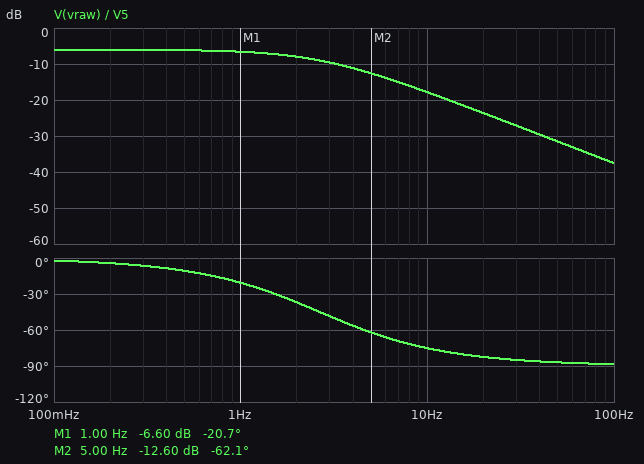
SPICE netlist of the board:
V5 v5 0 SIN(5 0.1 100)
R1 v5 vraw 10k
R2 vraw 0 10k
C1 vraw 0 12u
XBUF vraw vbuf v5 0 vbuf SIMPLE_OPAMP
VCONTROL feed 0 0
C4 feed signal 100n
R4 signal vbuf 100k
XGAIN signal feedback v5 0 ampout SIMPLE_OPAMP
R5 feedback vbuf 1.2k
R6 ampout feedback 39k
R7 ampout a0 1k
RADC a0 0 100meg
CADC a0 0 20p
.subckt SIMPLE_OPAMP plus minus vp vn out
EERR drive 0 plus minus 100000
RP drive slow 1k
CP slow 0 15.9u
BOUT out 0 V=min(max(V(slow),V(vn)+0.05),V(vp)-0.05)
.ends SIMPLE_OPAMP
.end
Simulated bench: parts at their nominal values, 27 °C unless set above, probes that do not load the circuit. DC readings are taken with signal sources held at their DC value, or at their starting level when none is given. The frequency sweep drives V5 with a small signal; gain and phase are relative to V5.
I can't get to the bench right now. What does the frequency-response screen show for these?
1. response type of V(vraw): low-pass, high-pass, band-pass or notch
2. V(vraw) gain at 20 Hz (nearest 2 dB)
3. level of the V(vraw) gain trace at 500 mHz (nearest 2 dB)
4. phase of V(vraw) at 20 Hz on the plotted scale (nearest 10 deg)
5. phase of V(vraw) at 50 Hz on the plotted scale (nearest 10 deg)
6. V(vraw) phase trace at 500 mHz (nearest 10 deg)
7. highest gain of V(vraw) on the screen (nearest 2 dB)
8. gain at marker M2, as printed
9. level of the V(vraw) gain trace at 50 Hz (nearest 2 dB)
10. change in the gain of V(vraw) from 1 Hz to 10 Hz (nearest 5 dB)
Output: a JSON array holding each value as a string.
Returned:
["low-pass", "-24 dB", "-6 dB", "-80 deg", "-90 deg", "-10 deg", "-6 dB", "-12.60 dB", "-32 dB", "-10 dB"]
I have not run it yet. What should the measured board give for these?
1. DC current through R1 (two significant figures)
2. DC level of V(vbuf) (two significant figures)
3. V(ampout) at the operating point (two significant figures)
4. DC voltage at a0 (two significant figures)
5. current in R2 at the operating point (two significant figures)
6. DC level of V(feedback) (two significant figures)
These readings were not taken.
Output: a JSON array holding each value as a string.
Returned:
["250 µA", "2.5 V", "2.5 V", "2.5 V", "250 µA", "2.5 V"]
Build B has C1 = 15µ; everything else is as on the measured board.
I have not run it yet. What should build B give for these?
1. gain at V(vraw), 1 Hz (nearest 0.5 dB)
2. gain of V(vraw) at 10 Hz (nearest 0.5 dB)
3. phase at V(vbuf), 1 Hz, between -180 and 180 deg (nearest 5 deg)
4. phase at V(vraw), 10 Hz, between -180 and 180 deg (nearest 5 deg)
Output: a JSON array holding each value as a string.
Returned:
["-7.0 dB", "-19.5 dB", "-25 deg", "-80 deg"]
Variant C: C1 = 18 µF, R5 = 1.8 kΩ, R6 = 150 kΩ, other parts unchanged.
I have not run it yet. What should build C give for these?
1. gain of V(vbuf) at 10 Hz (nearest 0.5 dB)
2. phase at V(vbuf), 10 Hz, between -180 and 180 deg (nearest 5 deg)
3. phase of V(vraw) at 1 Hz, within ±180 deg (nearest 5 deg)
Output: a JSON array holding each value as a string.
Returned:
["-21.0 dB", "-80 deg", "-30 deg"]
